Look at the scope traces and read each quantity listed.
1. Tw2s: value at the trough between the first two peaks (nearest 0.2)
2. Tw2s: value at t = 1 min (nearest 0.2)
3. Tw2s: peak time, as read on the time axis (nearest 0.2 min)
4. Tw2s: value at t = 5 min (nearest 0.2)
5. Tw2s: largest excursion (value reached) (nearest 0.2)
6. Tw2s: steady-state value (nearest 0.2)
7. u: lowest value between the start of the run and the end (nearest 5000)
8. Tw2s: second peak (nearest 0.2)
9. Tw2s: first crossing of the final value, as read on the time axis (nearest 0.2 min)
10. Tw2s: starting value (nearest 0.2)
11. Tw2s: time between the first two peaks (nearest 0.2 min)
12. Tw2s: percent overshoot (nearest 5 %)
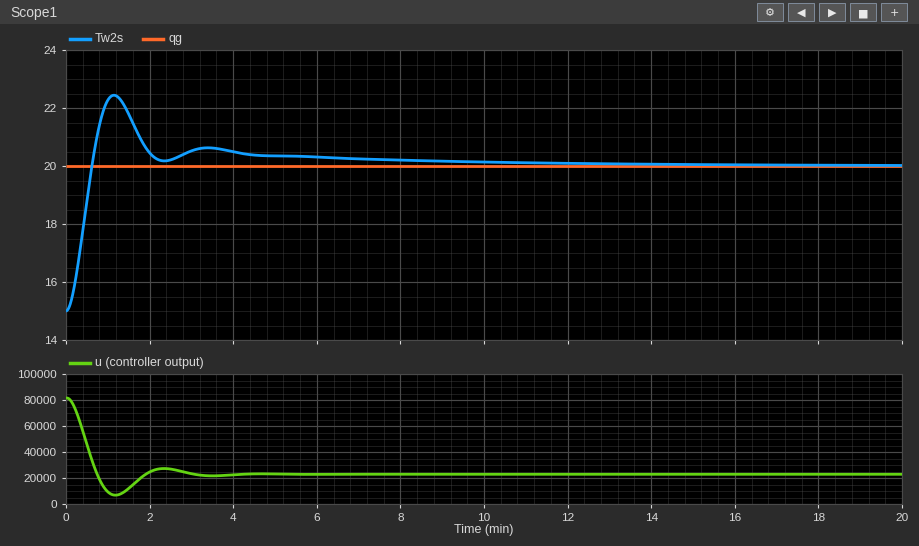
20.2
22.2
1.2 min
20.4
22.4
20.0
5000
20.6
0.6 min
15.0
2.2 min
50 %
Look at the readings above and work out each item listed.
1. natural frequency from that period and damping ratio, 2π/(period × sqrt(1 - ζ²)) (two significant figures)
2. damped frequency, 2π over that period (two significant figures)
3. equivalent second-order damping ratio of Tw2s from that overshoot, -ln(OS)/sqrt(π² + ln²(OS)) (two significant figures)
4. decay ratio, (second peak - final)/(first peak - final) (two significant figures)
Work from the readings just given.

2.9 rad/min
2.9 rad/min
0.22
0.25
